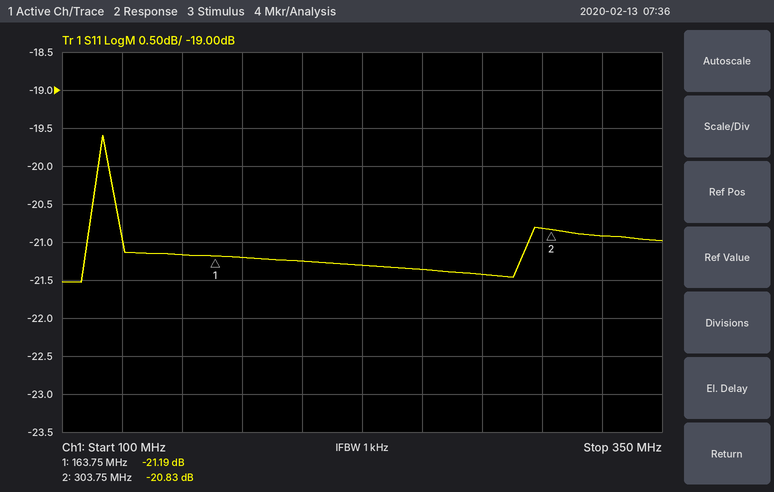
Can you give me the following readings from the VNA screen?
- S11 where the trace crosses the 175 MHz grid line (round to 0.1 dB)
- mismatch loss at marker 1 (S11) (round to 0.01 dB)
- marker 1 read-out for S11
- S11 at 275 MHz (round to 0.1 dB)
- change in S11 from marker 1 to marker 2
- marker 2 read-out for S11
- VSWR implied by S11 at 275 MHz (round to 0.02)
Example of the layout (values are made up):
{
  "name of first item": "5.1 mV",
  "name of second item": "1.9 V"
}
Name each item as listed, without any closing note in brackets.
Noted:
{
  "S11 where the trace crosses the 175 MHz grid line": "-21.2 dB",
  "mismatch loss at marker 1 (S11)": "0.03 dB",
  "marker 1 read-out for S11": "-21.19 dB",
  "S11 at 275 MHz": "-21.4 dB",
  "change in S11 from marker 1 to marker 2": "0.36 dB",
  "marker 2 read-out for S11": "-20.83 dB",
  "VSWR implied by S11 at 275 MHz": "1.18"
}
